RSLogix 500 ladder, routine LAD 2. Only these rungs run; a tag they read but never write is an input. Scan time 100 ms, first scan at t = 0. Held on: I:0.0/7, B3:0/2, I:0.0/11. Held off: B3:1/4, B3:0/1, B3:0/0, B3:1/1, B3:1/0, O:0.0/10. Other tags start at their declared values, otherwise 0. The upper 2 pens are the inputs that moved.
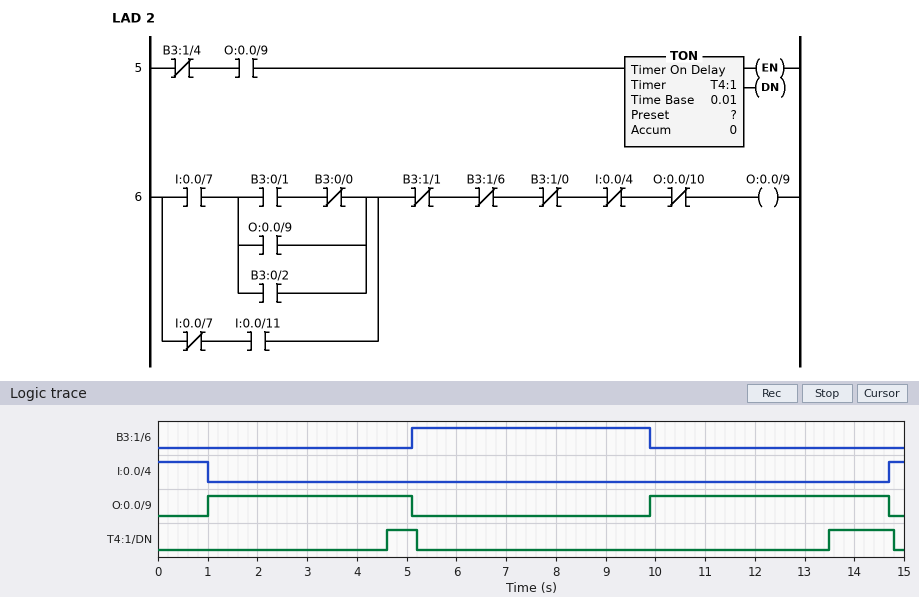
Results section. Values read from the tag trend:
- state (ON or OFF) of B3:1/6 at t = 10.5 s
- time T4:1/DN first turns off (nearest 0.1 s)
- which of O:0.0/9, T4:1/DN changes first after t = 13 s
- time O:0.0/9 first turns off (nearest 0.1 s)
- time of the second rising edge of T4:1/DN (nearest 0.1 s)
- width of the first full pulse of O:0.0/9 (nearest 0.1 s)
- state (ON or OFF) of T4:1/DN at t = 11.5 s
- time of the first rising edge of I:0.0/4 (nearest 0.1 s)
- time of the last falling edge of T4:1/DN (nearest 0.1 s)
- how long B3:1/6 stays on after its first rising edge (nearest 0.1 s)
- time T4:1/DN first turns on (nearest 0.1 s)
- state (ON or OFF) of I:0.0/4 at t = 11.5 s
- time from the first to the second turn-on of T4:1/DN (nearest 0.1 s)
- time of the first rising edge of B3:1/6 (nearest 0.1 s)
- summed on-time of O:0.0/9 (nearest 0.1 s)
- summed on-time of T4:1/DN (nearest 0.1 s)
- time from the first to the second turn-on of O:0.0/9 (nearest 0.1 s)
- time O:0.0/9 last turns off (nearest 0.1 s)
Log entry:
OFF
5.2 s
T4:1/DN
5.1 s
13.5 s
4.1 s
OFF
14.7 s
14.8 s
4.8 s
4.6 s
OFF
8.9 s
5.1 s
8.9 s
1.9 s
8.9 s
14.7 s
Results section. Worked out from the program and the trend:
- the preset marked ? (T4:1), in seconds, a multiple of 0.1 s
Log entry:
3.5 s
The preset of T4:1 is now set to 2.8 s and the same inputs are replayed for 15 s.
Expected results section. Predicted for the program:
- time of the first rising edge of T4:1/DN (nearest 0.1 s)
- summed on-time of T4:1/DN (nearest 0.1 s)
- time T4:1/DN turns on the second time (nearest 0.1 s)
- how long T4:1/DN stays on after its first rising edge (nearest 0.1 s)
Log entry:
3.9 s
3.3 s
12.8 s
1.3 s
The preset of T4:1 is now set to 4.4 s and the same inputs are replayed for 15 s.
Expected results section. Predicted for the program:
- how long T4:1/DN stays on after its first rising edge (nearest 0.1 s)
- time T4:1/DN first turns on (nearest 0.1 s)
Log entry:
0.4 s
14.4 s
